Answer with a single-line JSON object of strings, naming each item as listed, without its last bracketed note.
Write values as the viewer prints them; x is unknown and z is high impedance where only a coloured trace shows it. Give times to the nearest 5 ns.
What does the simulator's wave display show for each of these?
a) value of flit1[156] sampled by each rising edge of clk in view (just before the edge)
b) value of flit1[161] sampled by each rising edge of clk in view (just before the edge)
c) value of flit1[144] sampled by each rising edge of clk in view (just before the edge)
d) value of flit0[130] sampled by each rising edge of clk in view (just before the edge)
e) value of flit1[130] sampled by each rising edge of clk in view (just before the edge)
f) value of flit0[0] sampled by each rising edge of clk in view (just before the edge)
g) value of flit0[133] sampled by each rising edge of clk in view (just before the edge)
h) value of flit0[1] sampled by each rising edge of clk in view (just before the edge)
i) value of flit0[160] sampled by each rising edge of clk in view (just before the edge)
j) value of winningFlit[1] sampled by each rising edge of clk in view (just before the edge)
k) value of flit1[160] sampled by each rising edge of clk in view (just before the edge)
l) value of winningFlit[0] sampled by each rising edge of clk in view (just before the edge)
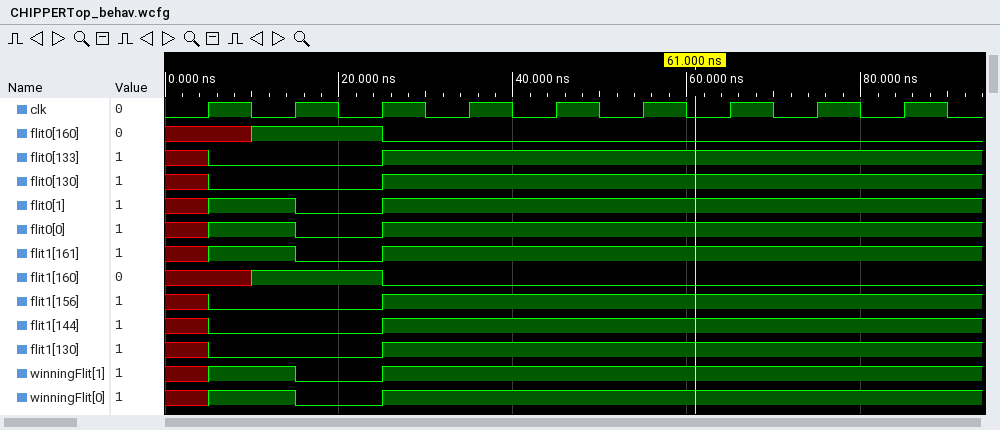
{"value of flit1[156] sampled by each rising edge of clk in view": "x 0 0 1 1 1 1 1 1", "value of flit1[161] sampled by each rising edge of clk in view": "x 1 0 1 1 1 1 1 1", "value of flit1[144] sampled by each rising edge of clk in view": "x 0 0 1 1 1 1 1 1", "value of flit0[130] sampled by each rising edge of clk in view": "x 0 0 1 1 1 1 1 1", "value of flit1[130] sampled by each rising edge of clk in view": "x 0 0 1 1 1 1 1 1", "value of flit0[0] sampled by each rising edge of clk in view": "x 1 0 1 1 1 1 1 1", "value of flit0[133] sampled by each rising edge of clk in view": "x 0 0 1 1 1 1 1 1", "value of flit0[1] sampled by each rising edge of clk in view": "x 1 0 1 1 1 1 1 1", "value of flit0[160] sampled by each rising edge of clk in view": "x 1 1 0 0 0 0 0 0", "value of winningFlit[1] sampled by each rising edge of clk in view": "x 1 0 1 1 1 1 1 1", "value of flit1[160] sampled by each rising edge of clk in view": "x 1 1 0 0 0 0 0 0", "value of winningFlit[0] sampled by each rising edge of clk in view": "x 1 0 1 1 1 1 1 1"}
